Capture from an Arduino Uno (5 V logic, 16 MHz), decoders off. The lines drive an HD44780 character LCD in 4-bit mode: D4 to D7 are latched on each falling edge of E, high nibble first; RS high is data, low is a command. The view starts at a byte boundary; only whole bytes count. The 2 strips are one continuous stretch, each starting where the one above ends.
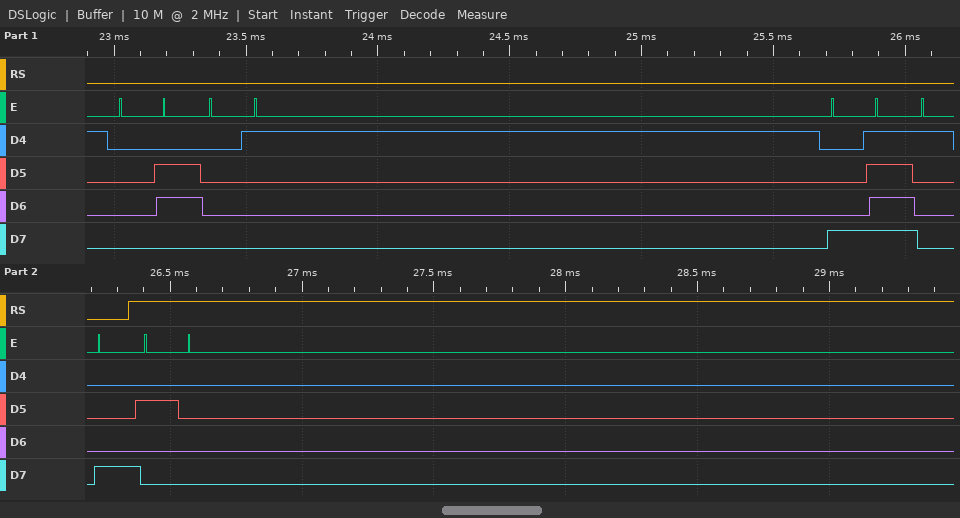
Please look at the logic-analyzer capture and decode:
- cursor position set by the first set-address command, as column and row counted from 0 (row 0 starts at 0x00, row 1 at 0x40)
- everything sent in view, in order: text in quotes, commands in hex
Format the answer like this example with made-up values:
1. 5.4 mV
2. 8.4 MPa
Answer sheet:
1. column 15, row 0
2. 0x06 0x01 0x8F 0x18 " "
